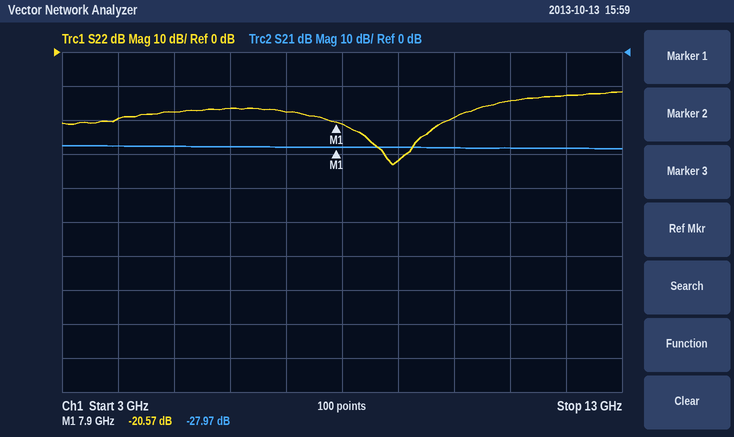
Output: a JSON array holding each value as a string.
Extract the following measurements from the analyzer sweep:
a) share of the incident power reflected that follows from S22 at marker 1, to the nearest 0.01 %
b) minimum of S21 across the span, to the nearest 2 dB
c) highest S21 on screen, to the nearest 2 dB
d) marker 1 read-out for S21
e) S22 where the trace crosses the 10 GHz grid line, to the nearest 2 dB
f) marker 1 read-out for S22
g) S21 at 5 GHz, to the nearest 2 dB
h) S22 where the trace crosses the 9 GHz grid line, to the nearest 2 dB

["0.88 %", "-28 dB", "-28 dB", "-27.97 dB", "-20 dB", "-20.57 dB", "-28 dB", "-32 dB"]
